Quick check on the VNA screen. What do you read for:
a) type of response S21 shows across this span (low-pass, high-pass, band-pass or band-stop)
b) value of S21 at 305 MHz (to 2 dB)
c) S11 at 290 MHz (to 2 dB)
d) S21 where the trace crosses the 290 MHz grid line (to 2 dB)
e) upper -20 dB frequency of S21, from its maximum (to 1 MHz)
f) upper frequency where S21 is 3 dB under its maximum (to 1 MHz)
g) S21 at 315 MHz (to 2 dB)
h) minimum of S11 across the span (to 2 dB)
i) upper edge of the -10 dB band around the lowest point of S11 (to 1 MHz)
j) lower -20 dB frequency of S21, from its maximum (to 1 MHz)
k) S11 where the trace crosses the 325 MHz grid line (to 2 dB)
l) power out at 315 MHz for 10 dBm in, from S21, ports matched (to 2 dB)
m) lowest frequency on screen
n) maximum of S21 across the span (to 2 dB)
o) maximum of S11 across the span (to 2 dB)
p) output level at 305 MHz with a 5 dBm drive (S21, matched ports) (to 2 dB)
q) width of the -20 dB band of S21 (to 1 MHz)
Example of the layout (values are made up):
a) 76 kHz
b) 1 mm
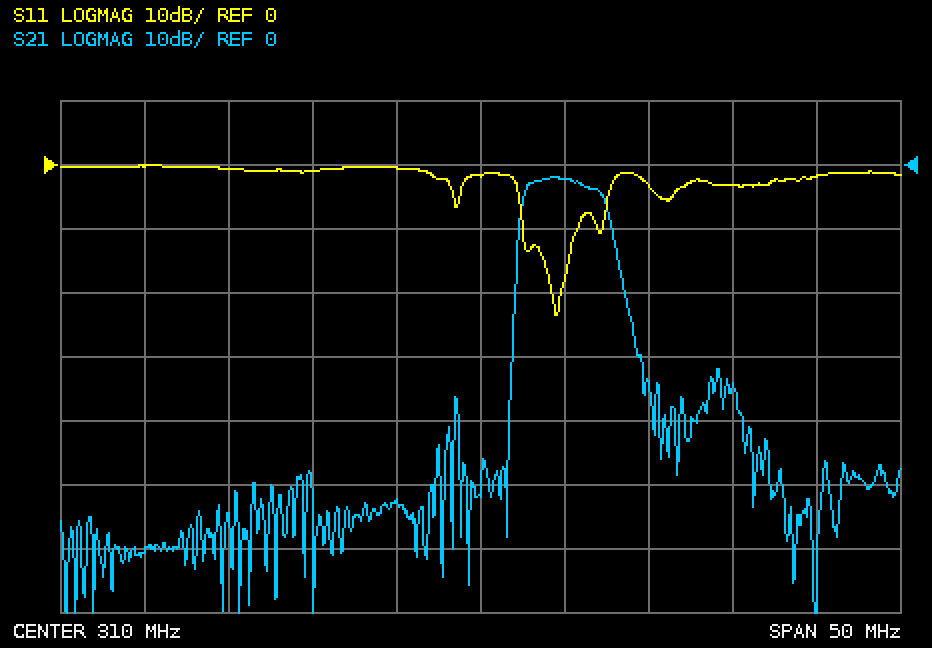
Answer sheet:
a) band-pass
b) -52 dB
c) 0 dB
d) -60 dB
e) 319 MHz
f) 317 MHz
g) -2 dB
h) -24 dB
i) 316 MHz
j) 312 MHz
k) -4 dB
l) 8 dBm
m) 285 MHz
n) -2 dB
o) 0 dB
p) -48 dBm
q) 7 MHz
